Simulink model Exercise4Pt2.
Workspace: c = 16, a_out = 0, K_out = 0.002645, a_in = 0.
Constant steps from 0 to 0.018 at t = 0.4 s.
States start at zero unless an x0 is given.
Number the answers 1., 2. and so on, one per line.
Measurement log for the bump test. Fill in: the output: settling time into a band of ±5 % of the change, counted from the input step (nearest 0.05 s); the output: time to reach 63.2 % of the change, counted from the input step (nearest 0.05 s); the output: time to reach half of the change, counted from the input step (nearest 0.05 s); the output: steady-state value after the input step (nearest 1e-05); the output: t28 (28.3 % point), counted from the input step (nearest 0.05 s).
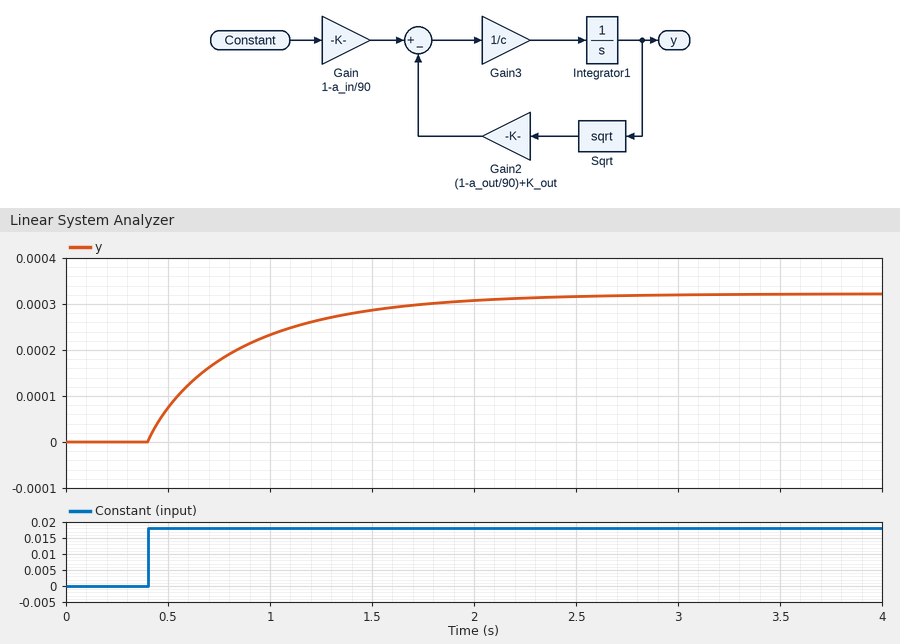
1. 1.55 s
2. 0.45 s
3. 0.30 s
4. 0.00032
5. 0.15 s
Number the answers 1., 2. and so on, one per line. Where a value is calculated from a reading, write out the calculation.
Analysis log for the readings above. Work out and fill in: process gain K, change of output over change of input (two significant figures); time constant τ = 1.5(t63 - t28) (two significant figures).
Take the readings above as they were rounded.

1. (0.00032 - 0) / 0.018 = 0.018
2. 1.5 × (0.45 - 0.15) = 0.45 s
